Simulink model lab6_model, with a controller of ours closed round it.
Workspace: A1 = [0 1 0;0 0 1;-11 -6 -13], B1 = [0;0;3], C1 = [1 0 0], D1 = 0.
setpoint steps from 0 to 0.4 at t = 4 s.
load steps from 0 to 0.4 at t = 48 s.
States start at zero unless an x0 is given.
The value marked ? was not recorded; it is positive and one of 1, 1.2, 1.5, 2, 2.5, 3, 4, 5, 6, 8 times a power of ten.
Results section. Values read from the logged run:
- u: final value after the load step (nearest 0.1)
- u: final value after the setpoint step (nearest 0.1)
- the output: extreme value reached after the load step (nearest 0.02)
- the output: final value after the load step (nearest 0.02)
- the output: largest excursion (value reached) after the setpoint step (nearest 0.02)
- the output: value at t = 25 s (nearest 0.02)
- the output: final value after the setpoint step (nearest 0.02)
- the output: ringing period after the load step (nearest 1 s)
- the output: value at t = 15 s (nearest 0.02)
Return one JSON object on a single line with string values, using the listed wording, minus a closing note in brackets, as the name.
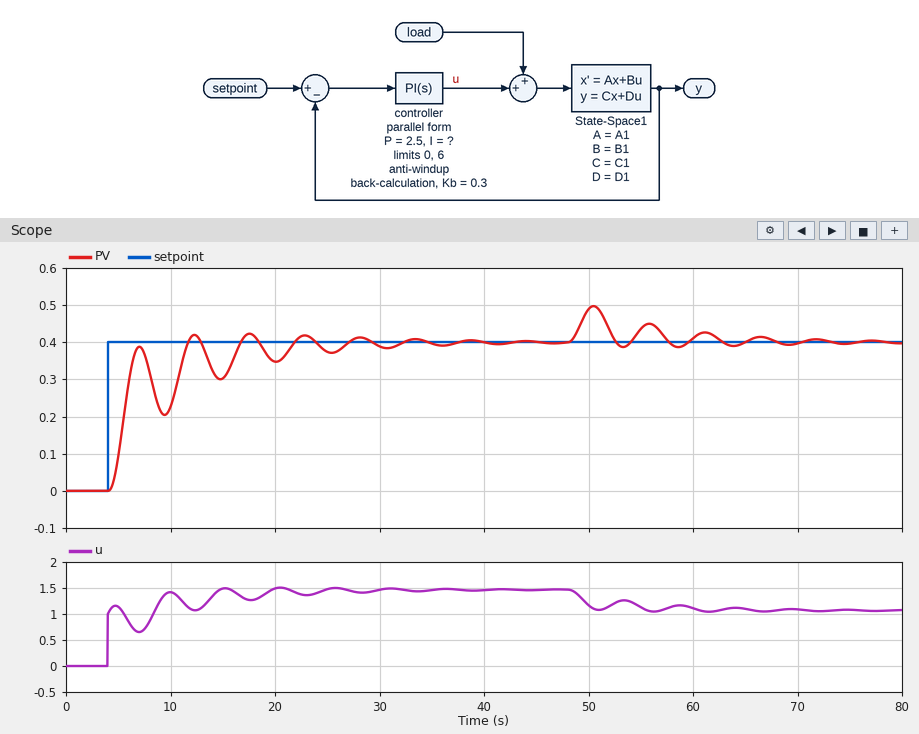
{"u: final value after the load step": "1.1", "u: final value after the setpoint step": "1.5", "the output: extreme value reached after the load step": "0.50", "the output: final value after the load step": "0.40", "the output: largest excursion (value reached) after the setpoint step": "0.42", "the output: value at t = 25 s": "0.38", "the output: final value after the setpoint step": "0.40", "the output: ringing period after the load step": "5 s", "the output: value at t = 15 s": "0.30"}
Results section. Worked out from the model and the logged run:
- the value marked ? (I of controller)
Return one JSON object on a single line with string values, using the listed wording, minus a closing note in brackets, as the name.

{"the value marked ?": "1"}
